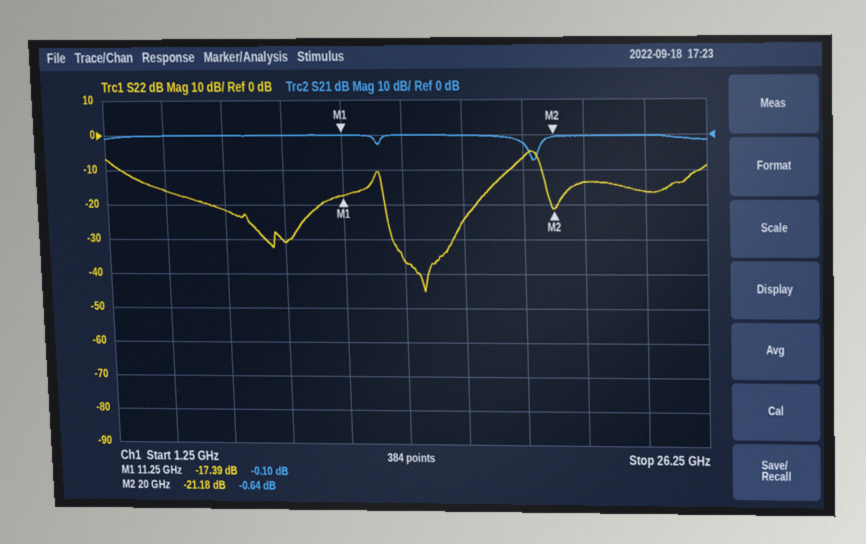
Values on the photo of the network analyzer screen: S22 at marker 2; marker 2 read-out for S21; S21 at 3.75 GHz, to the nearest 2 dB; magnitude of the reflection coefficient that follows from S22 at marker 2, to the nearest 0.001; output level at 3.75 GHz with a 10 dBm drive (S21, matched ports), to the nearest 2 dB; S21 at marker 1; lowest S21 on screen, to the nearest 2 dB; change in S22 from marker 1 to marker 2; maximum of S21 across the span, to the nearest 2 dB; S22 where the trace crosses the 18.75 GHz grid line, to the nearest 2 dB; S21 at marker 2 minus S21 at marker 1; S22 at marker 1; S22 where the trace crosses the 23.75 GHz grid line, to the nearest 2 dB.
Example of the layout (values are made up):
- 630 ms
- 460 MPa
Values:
- -21.18 dB
- -0.64 dB
- 0 dB
- 0.087
- 10 dBm
- -0.10 dB
- -8 dB
- -3.79 dB
- 0 dB
- -6 dB
- -0.54 dB
- -17.39 dB
- -16 dB
